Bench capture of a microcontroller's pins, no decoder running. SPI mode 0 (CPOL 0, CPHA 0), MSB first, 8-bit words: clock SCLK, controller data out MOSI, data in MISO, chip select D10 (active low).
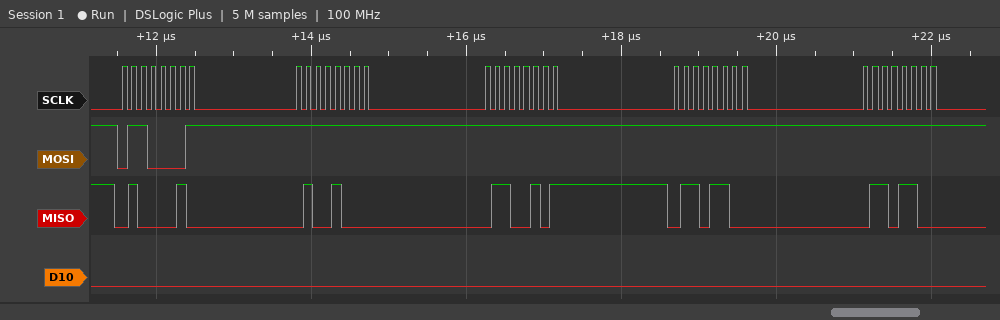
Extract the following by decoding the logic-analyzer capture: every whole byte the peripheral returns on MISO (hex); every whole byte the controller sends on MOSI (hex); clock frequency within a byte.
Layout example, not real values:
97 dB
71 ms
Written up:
0x42 0x48 0x65 0x6C 0x6C
0x61 0xFF 0xFF 0xFF 0xFF
8 MHz
